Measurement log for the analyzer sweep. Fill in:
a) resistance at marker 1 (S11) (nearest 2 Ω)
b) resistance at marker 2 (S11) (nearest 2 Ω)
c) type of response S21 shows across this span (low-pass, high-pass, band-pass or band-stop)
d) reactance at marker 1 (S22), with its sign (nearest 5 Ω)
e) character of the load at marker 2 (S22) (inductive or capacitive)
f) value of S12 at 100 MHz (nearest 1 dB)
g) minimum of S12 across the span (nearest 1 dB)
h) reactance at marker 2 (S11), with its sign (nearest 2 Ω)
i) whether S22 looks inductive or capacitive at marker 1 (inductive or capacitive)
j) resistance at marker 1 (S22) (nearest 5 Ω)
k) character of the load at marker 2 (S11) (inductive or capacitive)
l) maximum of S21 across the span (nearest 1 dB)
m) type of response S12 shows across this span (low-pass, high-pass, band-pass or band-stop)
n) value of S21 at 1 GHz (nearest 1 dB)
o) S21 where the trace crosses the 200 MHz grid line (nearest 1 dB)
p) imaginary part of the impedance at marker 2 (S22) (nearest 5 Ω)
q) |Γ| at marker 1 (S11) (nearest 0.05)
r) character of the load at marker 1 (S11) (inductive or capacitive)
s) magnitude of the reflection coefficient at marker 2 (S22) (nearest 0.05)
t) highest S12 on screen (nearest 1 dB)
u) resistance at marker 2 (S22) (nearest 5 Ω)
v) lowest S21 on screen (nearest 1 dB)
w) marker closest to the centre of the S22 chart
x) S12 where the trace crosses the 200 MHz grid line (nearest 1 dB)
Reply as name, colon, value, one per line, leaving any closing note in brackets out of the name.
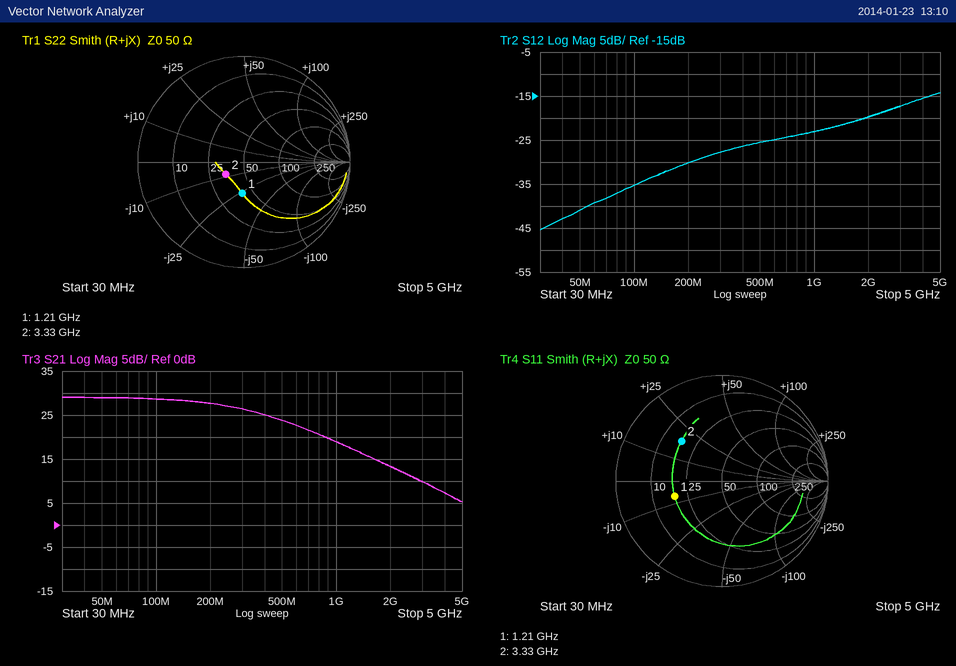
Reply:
resistance at marker 1 (S11): 18 Ω
resistance at marker 2 (S11): 18 Ω
type of response S21 shows across this span: low-pass
reactance at marker 1 (S22), with its sign: -25 Ω
character of the load at marker 2 (S22): capacitive
value of S12 at 100 MHz: -35 dB
minimum of S12 across the span: -45 dB
reactance at marker 2 (S11), with its sign: +18 Ω
whether S22 looks inductive or capacitive at marker 1: capacitive
resistance at marker 1 (S22): 40 Ω
character of the load at marker 2 (S11): inductive
maximum of S21 across the span: 29 dB
type of response S12 shows across this span: high-pass
value of S21 at 1 GHz: 19 dB
S21 where the trace crosses the 200 MHz grid line: 28 dB
imaginary part of the impedance at marker 2 (S22): -10 Ω
|Γ| at marker 1 (S11): 0.45
character of the load at marker 1 (S11): capacitive
magnitude of the reflection coefficient at marker 2 (S22): 0.20
highest S12 on screen: -14 dB
resistance at marker 2 (S22): 35 Ω
lowest S21 on screen: 5 dB
marker closest to the centre of the S22 chart: marker 2
S12 where the trace crosses the 200 MHz grid line: -30 dB
